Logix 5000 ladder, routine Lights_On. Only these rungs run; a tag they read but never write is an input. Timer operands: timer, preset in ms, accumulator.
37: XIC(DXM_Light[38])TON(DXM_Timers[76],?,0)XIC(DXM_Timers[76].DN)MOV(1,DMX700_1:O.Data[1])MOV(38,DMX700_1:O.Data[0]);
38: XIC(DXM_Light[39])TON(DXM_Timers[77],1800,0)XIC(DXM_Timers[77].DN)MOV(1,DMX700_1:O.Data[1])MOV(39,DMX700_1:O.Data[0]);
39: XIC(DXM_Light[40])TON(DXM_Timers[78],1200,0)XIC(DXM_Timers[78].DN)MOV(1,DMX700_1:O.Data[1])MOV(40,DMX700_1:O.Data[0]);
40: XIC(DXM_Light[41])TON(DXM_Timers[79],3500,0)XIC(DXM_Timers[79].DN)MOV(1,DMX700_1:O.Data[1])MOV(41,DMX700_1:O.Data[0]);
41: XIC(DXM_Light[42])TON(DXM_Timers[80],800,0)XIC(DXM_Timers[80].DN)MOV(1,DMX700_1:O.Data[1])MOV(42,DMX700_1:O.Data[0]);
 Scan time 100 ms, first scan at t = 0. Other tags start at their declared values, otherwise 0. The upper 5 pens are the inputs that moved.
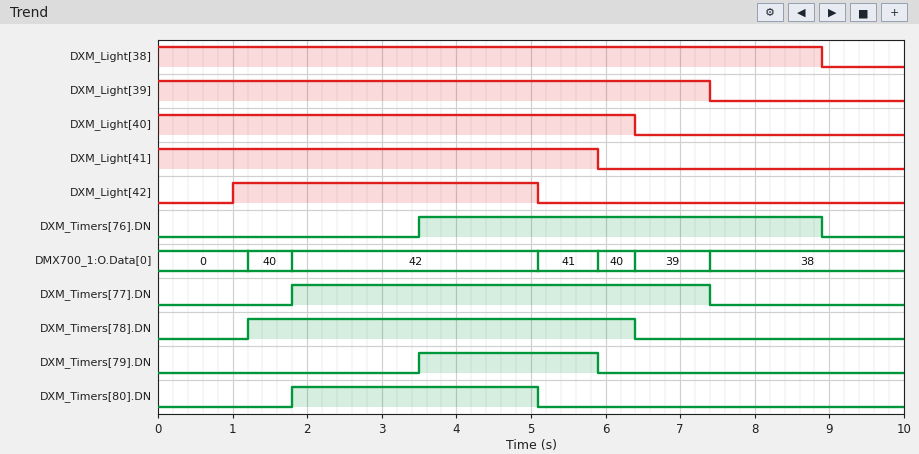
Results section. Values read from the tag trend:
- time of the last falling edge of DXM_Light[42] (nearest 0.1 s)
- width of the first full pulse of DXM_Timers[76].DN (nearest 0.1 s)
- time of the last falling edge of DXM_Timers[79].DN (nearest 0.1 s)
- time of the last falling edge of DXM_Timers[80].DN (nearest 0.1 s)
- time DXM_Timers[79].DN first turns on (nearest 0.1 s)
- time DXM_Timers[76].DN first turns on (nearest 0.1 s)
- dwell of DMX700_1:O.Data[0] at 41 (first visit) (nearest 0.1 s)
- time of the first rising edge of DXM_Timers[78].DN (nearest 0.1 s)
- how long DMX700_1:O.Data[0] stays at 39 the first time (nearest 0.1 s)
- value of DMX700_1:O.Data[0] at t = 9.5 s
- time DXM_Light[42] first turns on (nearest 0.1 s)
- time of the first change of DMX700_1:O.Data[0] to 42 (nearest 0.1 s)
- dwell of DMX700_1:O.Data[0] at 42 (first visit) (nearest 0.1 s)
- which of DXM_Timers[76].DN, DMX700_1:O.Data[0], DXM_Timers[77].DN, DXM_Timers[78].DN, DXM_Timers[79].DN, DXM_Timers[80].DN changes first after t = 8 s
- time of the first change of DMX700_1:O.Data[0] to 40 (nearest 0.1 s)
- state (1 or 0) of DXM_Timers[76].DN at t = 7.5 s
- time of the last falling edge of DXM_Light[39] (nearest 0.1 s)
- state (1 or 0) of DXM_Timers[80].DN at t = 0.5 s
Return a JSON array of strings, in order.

["5.1 s", "5.4 s", "5.9 s", "5.1 s", "3.5 s", "3.5 s", "0.8 s", "1.2 s", "1.0 s", "38", "1.0 s", "1.8 s", "3.3 s", "DXM_Timers[76].DN", "1.2 s", "1", "7.4 s", "0"]
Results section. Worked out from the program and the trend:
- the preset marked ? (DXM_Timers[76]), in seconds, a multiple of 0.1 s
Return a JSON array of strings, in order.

["3.5 s"]
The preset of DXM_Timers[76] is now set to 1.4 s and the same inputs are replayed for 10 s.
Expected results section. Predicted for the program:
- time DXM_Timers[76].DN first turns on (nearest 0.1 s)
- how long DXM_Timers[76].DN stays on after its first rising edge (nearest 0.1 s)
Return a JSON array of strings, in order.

["1.4 s", "7.5 s"]
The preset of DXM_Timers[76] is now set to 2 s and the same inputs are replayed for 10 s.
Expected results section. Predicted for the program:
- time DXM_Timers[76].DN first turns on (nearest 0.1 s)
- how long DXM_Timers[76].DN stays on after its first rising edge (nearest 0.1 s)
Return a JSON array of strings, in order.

["2.0 s", "6.9 s"]
